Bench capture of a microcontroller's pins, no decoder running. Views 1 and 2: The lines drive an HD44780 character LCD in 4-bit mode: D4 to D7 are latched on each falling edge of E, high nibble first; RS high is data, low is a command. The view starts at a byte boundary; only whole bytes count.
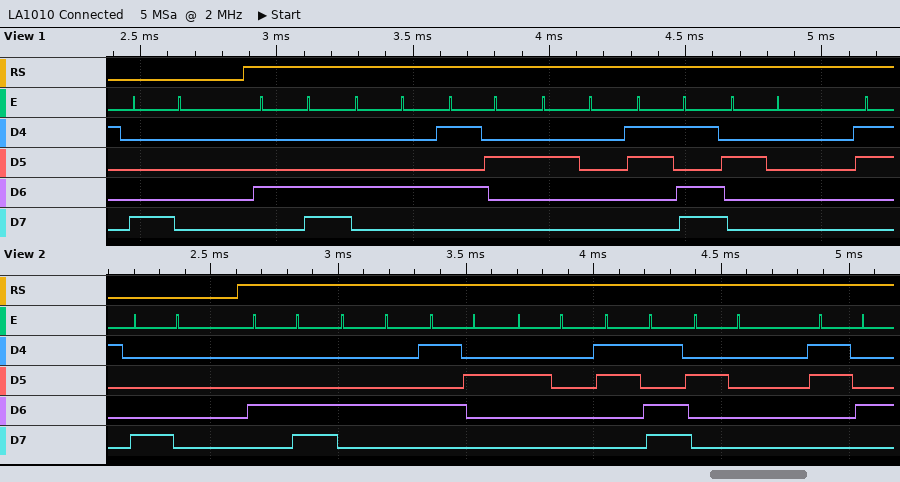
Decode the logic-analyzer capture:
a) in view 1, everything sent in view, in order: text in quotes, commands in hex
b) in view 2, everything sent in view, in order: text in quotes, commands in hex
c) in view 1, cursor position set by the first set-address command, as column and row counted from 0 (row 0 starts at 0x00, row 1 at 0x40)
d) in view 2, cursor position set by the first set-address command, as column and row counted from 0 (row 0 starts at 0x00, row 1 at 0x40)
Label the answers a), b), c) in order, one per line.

a) 0x80 "LDR = "
b) 0x80 "LDR = 4"
c) column 0, row 0
d) column 0, row 0
